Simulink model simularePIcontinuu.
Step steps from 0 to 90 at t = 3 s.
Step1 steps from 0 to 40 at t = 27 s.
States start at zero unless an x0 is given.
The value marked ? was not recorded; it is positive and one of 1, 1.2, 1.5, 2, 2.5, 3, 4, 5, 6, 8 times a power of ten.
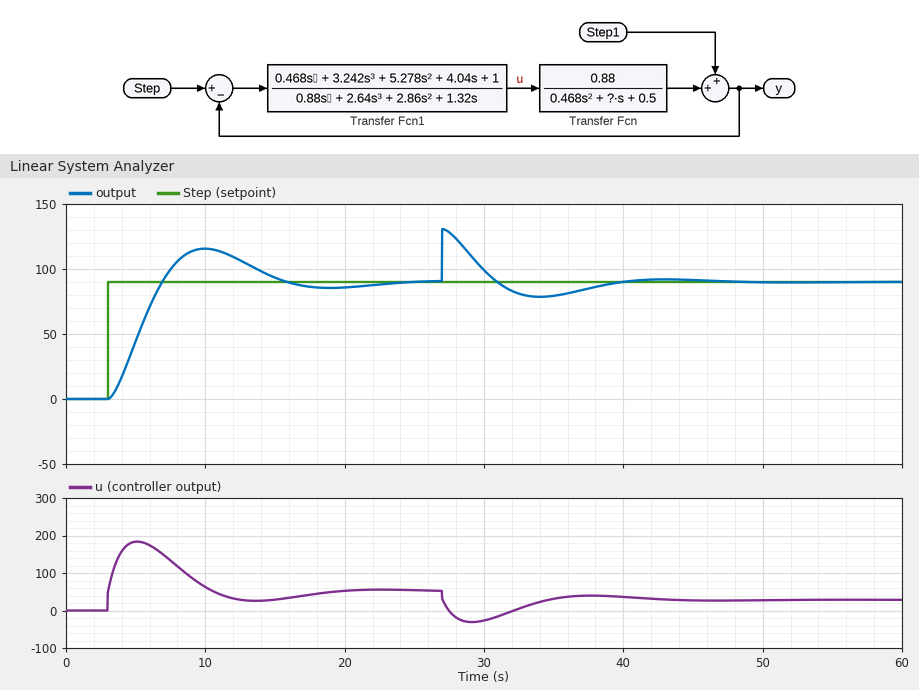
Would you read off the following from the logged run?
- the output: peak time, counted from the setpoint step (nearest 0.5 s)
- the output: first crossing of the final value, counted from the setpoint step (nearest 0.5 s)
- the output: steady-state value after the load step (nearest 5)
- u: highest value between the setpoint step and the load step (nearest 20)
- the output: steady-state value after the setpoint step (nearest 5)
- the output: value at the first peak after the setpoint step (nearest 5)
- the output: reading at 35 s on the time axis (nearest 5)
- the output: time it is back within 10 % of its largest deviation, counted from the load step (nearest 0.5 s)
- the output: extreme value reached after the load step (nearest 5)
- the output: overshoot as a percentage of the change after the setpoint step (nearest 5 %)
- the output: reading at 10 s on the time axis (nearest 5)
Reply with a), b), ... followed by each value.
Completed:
a) 7.0 s
b) 4.0 s
c) 90
d) 180
e) 90
f) 115
g) 80
h) 11.0 s
i) 130
j) 30 %
k) 115
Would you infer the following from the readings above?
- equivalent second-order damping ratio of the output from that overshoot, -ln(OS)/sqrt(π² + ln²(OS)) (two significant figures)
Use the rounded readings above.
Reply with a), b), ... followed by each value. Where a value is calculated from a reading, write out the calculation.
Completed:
a) ln(0.3) = -1.204; 1.204 / sqrt(9.870 + 1.450) = 0.36
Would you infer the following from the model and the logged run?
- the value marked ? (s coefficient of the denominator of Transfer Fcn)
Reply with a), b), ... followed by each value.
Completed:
a) 5
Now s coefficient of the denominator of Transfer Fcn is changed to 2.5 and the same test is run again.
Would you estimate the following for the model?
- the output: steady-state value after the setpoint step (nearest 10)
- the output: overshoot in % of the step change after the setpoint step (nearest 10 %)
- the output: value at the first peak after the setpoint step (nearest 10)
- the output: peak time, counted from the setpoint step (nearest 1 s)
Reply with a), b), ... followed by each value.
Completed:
a) 90
b) 20 %
c) 110
d) 4 s
